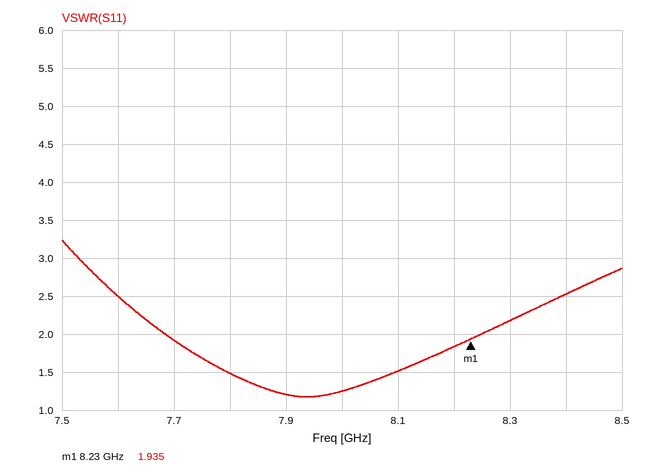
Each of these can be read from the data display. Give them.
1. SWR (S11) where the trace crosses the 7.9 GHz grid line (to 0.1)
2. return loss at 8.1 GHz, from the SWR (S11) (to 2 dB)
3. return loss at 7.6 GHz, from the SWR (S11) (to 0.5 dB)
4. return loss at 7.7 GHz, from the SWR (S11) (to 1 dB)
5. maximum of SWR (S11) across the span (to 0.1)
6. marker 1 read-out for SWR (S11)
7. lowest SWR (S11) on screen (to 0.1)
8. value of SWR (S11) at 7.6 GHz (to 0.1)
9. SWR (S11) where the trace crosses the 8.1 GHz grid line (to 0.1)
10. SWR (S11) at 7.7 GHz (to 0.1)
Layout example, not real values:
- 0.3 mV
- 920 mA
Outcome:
- 1.2
- 14 dB
- 7.5 dB
- 10 dB
- 3.2
- 1.935
- 1.2
- 2.5
- 1.5
- 1.9
